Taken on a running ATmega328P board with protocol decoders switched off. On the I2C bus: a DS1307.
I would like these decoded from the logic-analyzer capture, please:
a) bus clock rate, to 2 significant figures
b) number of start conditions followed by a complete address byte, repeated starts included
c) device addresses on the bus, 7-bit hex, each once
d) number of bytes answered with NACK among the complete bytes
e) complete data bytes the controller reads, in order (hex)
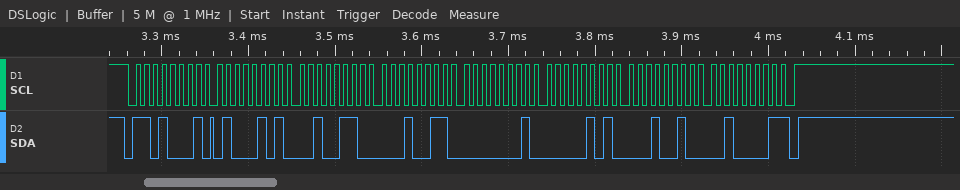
100 kHz
1
0x68
1
45 26 13 01 05 12 21
